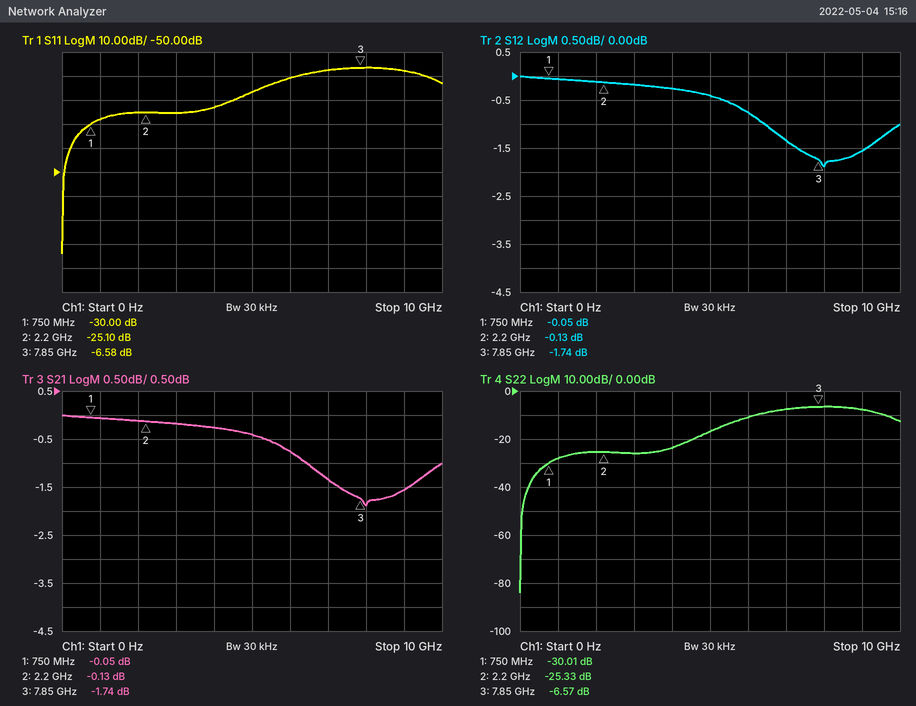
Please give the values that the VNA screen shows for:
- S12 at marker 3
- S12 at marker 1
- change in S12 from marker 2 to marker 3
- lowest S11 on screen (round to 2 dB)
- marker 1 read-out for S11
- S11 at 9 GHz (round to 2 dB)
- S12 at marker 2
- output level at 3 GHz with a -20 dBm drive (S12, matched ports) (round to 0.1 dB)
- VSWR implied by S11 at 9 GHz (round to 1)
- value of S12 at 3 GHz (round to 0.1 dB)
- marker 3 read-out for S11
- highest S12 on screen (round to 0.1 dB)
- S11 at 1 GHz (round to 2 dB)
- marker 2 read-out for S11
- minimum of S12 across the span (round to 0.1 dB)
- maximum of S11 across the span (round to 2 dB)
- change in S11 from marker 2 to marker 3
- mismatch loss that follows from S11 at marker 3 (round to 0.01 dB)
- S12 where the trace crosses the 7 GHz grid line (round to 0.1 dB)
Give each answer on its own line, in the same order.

-1.74 dB
-0.05 dB
-1.61 dB
-84 dB
-30.00 dB
-8 dB
-0.13 dB
-20.2 dBm
2
-0.2 dB
-6.58 dB
0.0 dB
-28 dB
-25.10 dB
-1.9 dB
-6 dB
18.52 dB
1.08 dB
-1.3 dB
